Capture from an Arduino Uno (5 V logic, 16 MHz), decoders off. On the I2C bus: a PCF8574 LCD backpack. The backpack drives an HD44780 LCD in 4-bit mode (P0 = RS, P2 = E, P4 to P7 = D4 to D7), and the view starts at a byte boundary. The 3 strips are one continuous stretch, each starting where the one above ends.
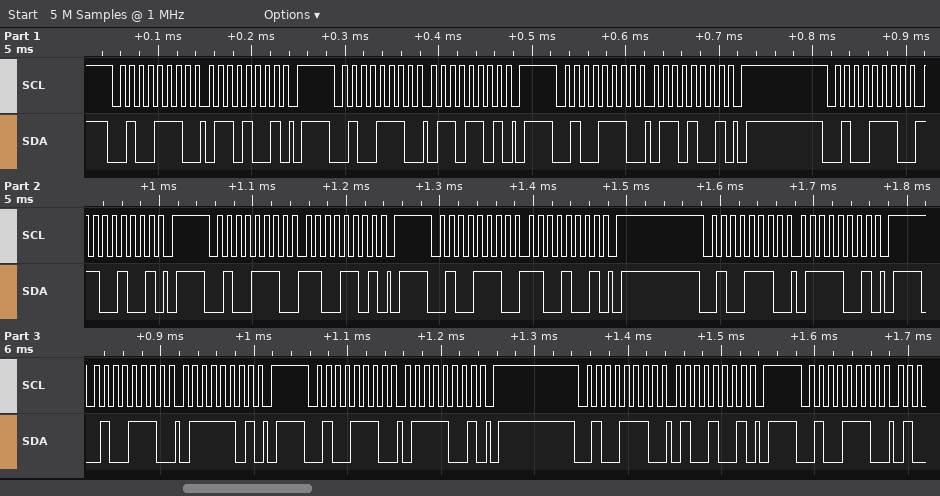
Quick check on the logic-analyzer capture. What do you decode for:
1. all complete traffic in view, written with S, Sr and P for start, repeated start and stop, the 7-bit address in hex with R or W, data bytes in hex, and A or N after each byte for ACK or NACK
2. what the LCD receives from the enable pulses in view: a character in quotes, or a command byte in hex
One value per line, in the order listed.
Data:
S 27W A 69 A P S 27W A 6D A P S 27W A 69 A P S 27W A C9 A P S 27W A CD A P S 27W A C9 A P S 27W A 79 A P S 27W A 7D A P S 27W A 79 A P S 27W A 49 A P S 27W A
'l'
